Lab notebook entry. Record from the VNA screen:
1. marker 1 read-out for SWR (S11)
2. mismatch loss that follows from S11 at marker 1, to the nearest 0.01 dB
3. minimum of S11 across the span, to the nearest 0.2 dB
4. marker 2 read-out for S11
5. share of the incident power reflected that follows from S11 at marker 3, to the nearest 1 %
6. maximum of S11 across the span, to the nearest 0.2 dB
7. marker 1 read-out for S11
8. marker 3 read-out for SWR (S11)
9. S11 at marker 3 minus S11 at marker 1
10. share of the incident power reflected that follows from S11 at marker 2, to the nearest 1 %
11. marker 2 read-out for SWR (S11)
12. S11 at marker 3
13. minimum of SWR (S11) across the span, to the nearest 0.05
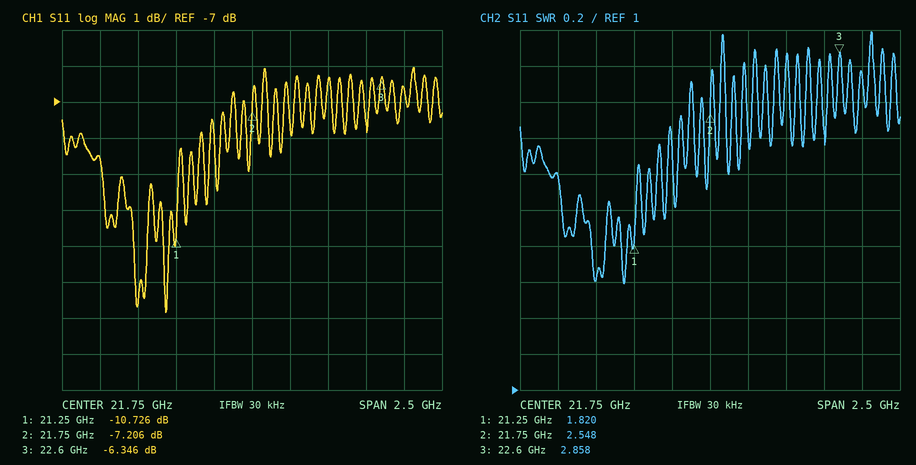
1.820
0.38 dB
-12.8 dB
-7.206 dB
23 %
-6.0 dB
-10.726 dB
2.858
4.380 dB
19 %
2.548
-6.346 dB
1.60
